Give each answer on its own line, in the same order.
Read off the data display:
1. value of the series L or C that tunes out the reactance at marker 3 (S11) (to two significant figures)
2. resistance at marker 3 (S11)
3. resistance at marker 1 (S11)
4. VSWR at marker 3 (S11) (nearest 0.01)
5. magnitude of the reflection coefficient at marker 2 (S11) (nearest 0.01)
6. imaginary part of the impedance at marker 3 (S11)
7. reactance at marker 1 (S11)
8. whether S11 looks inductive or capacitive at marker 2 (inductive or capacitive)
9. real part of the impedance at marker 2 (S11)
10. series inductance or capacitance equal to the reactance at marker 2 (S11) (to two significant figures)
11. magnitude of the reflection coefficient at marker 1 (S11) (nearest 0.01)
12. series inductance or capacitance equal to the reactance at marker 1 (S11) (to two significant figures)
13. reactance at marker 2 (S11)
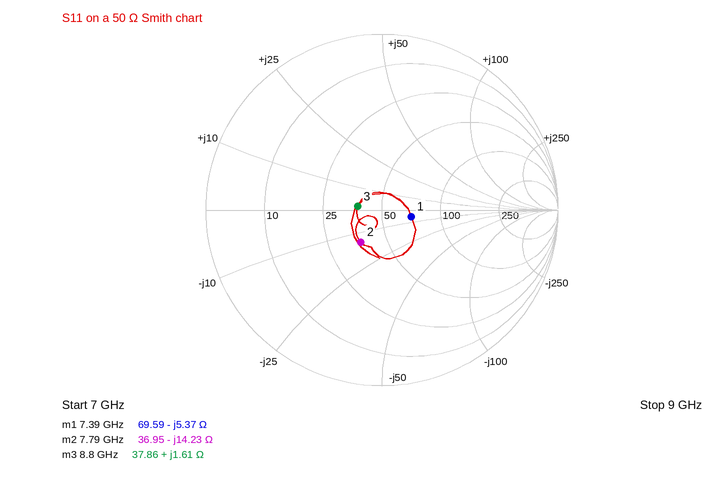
11 pF
37.86 Ω
69.59 Ω
1.32
0.22
+1.61 Ω
-5.37 Ω
capacitive
36.95 Ω
1.4 pF
0.17
4.0 pF
-14.23 Ω
